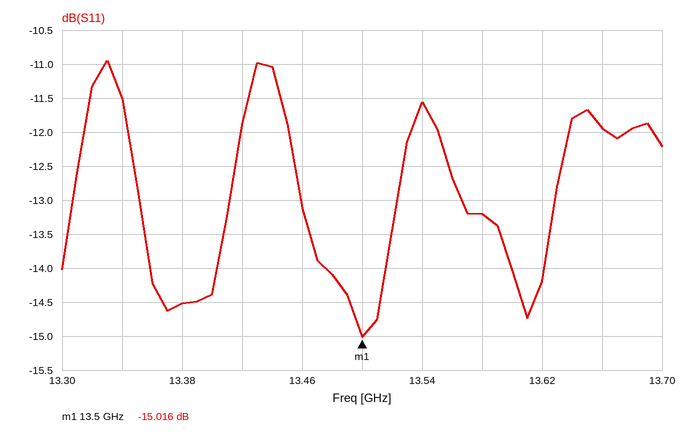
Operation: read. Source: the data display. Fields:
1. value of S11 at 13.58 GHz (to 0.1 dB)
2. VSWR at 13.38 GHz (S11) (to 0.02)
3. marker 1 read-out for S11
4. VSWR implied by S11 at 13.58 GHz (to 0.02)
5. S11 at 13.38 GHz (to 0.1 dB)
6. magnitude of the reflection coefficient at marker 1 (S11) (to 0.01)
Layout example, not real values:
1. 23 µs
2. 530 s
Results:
1. -13.2 dB
2. 1.46
3. -15.016 dB
4. 1.56
5. -14.5 dB
6. 0.18
